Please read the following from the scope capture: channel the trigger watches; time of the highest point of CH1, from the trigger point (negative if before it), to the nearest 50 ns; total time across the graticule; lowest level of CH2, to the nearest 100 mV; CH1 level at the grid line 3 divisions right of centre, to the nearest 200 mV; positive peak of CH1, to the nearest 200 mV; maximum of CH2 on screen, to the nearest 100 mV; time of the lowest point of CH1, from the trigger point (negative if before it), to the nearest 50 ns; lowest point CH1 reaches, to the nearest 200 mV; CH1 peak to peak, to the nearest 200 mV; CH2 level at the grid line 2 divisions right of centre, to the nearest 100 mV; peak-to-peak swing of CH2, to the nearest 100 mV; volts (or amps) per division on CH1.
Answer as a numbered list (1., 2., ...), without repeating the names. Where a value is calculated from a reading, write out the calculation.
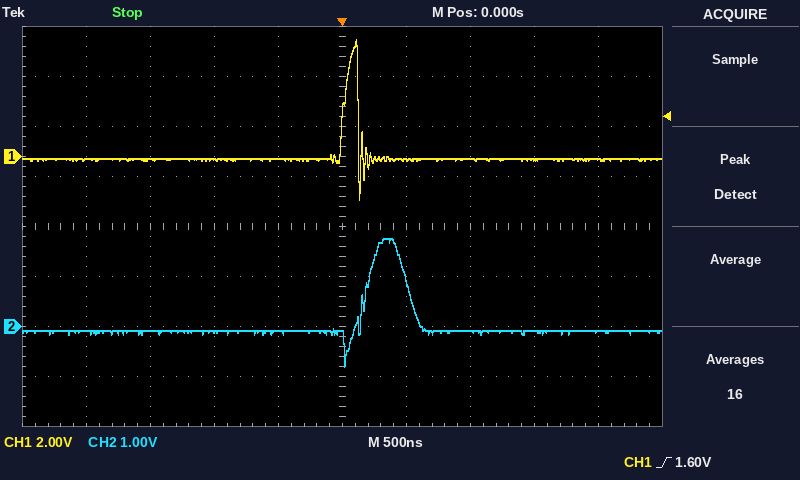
1. CH1
2. +100 ns
3. 5 µs
4. -800 mV
5. -200 mV
6. 4.6 V
7. 1.8 V
8. +150 ns
9. -1.8 V
10. 4.6 V − (-1.8 V) = 6.4 V
11. -100 mV
12. 1.8 V − (-800 mV) = 2.6 V
13. 2 V
